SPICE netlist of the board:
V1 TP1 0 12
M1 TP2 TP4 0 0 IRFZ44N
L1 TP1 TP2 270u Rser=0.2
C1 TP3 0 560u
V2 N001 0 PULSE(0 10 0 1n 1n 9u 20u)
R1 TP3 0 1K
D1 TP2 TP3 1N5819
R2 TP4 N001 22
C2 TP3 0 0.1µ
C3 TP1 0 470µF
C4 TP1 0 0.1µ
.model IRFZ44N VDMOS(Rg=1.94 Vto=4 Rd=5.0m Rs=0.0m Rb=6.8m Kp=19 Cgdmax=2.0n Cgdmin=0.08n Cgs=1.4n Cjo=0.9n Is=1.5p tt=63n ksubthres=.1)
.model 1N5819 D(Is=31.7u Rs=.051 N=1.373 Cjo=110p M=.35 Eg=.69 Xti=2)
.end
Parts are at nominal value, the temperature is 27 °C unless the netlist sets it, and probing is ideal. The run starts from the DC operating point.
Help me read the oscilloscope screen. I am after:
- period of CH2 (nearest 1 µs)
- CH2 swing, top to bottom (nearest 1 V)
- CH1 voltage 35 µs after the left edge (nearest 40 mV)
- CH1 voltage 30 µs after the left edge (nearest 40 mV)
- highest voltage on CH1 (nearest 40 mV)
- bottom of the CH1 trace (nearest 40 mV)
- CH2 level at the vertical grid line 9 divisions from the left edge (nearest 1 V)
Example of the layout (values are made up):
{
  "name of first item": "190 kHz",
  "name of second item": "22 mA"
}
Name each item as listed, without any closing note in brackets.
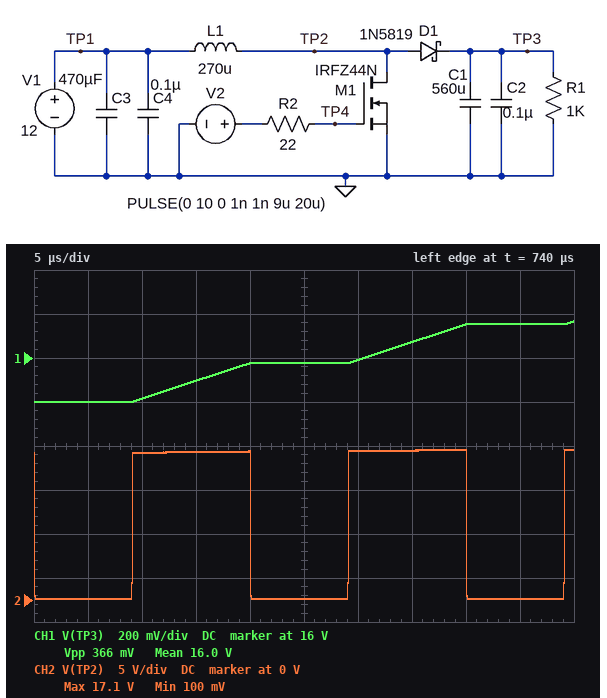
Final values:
{
  "period of CH2": "20 µs",
  "CH2 swing, top to bottom": "17 V",
  "CH1 voltage 35 µs after the left edge": "16.08 V",
  "CH1 voltage 30 µs after the left edge": "16.00 V",
  "highest voltage on CH1": "16.16 V",
  "bottom of the CH1 trace": "15.80 V",
  "CH2 level at the vertical grid line 9 divisions from the left edge": "0 V"
}
